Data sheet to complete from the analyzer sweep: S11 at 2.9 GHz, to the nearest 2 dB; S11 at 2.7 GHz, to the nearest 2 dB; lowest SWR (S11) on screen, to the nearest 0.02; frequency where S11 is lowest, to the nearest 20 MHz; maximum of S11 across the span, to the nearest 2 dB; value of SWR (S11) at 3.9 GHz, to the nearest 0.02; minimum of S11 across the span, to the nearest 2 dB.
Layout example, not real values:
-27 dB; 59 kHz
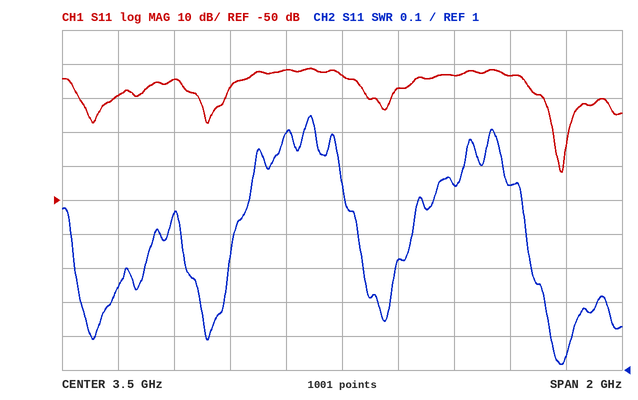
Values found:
-14 dB; -20 dB; 1.02; 4.28 GHz; -12 dB; 1.54; -42 dB
